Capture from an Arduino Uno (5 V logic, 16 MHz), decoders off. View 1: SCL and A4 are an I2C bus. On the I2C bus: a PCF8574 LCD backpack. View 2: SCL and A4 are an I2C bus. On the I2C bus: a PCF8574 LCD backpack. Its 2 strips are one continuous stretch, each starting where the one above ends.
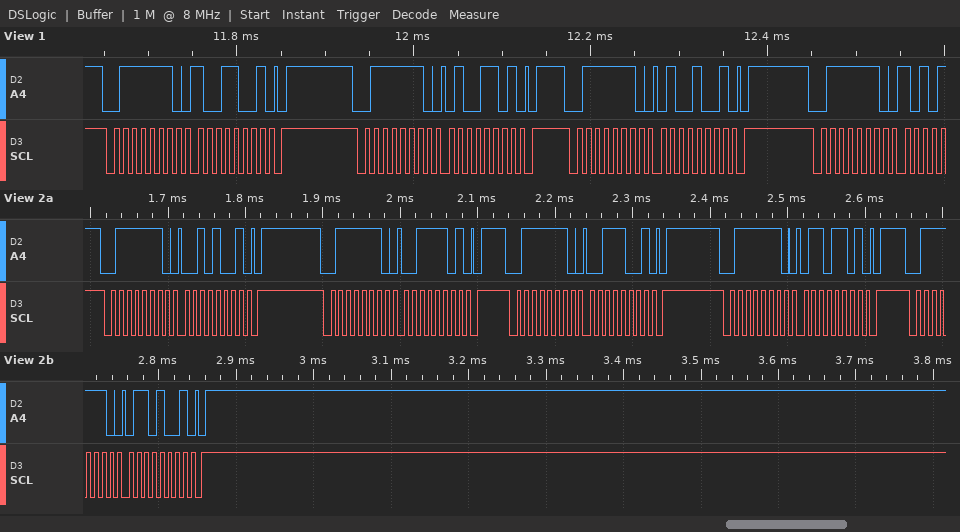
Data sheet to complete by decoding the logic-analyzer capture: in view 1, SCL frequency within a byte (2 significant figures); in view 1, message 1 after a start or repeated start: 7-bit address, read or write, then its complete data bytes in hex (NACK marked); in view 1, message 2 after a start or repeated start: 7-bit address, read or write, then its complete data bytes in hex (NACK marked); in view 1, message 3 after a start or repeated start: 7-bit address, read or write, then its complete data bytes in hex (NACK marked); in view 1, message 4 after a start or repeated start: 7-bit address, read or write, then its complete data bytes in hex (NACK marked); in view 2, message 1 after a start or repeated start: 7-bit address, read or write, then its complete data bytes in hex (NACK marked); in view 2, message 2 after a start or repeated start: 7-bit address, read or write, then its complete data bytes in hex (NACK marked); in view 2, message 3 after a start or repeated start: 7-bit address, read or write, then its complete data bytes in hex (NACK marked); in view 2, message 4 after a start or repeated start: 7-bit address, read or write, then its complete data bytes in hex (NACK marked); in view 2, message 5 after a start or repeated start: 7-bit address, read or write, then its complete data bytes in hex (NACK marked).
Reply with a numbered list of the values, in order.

1. 100 kHz
2. 0x3F write: 99
3. 0x3F write: 4D
4. 0x3F write: 49
5. 0x3F write
6. 0x3F write: 29
7. 0x3F write: 3D
8. 0x3F write: 39
9. 0x3F write: 6D
10. 0x3F write: 69
